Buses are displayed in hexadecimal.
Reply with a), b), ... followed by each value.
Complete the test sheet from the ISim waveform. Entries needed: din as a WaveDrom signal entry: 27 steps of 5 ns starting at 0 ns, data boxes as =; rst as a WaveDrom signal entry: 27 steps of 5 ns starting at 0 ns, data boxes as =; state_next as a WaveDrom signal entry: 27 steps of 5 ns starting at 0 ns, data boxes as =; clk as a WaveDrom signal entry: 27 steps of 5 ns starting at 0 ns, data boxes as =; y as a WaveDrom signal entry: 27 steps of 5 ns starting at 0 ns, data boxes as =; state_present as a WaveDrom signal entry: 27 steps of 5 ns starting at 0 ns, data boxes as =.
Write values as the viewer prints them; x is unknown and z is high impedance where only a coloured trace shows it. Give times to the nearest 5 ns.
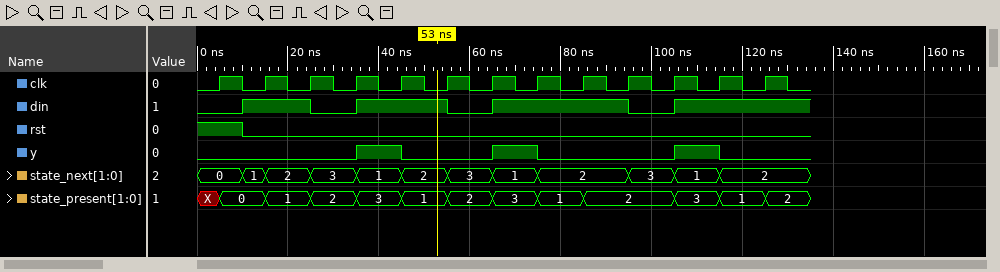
a) {name: 'din', wave: '0.1..0.1...0.1.....0.1.....'}
b) {name: 'rst', wave: '1.0........................'}
c) {name: 'state_next', wave: '=.==.=.=.=.=.=.=...=.=.=...', data: '0 1 2 3 1 2 3 1 2 3 1 2'}
d) {name: 'clk', wave: '010101010101010101010101010'}
e) {name: 'y', wave: '0......1.0...1.0.....1.0...'}
f) {name: 'state_present', wave: 'x=.=.=.=.=.=.=.=.=...=.=.=.', data: '0 1 2 3 1 2 3 1 2 3 1 2'}
